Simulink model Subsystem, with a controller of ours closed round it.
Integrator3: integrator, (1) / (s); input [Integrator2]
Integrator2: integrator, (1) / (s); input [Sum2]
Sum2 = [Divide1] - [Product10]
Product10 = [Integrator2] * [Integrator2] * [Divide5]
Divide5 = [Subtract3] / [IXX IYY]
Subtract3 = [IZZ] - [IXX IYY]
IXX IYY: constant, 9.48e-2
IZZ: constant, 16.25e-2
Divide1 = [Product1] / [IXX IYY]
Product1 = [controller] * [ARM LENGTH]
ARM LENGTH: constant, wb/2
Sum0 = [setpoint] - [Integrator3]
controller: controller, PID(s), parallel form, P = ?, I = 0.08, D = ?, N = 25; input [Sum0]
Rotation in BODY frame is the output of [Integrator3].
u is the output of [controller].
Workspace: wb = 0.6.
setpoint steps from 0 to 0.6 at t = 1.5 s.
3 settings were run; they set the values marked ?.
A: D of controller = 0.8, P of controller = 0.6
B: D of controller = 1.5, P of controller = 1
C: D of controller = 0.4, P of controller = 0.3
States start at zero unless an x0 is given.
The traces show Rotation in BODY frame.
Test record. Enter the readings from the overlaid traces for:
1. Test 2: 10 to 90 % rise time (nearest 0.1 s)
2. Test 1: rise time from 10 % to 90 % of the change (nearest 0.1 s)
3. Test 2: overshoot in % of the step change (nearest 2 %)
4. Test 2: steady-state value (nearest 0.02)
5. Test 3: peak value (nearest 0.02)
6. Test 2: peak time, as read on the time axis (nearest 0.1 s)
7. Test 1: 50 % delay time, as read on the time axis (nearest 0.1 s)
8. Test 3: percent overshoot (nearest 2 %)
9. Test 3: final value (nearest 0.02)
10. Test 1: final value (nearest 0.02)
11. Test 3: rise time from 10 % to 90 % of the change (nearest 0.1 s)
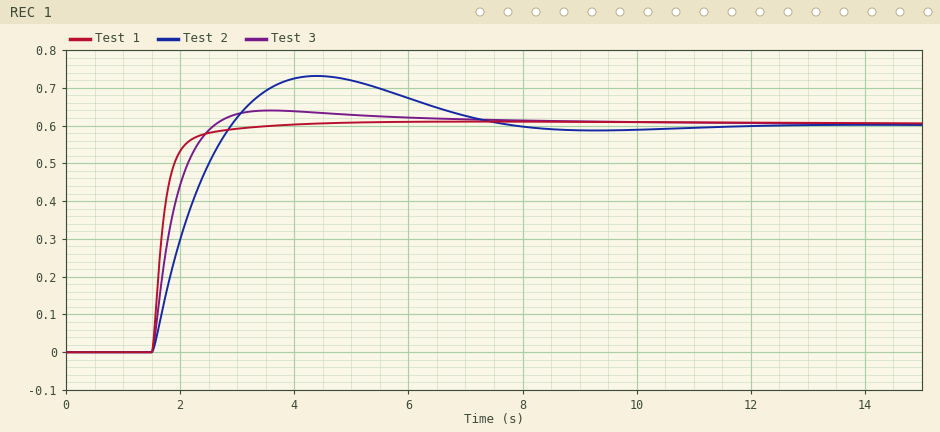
1.0 s
0.5 s
22 %
0.60
0.64
4.4 s
1.7 s
6 %
0.60
0.60
0.7 s
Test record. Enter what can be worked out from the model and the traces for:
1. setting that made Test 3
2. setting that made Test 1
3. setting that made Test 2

A
B
C
